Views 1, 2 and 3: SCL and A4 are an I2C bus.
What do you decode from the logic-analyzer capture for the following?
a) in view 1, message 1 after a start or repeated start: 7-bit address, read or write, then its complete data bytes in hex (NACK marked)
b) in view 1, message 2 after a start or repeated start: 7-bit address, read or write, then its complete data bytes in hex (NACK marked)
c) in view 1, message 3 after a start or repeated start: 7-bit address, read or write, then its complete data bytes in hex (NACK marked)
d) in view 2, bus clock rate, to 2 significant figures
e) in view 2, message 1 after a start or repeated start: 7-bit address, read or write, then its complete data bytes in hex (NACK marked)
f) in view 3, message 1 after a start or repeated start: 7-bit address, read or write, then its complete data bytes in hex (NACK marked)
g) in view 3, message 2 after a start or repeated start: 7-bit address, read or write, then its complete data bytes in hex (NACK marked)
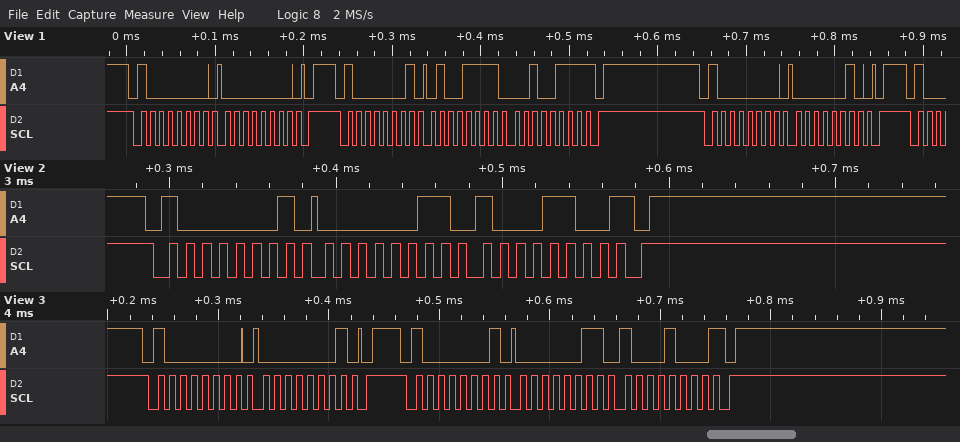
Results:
0x40 write: 00
0x40 read: 4F 27 NACK
0x40 write: 02
100 kHz
0x40 read: 03 8C NACK
0x40 write: 01
0x40 read: 03 88 NACK
